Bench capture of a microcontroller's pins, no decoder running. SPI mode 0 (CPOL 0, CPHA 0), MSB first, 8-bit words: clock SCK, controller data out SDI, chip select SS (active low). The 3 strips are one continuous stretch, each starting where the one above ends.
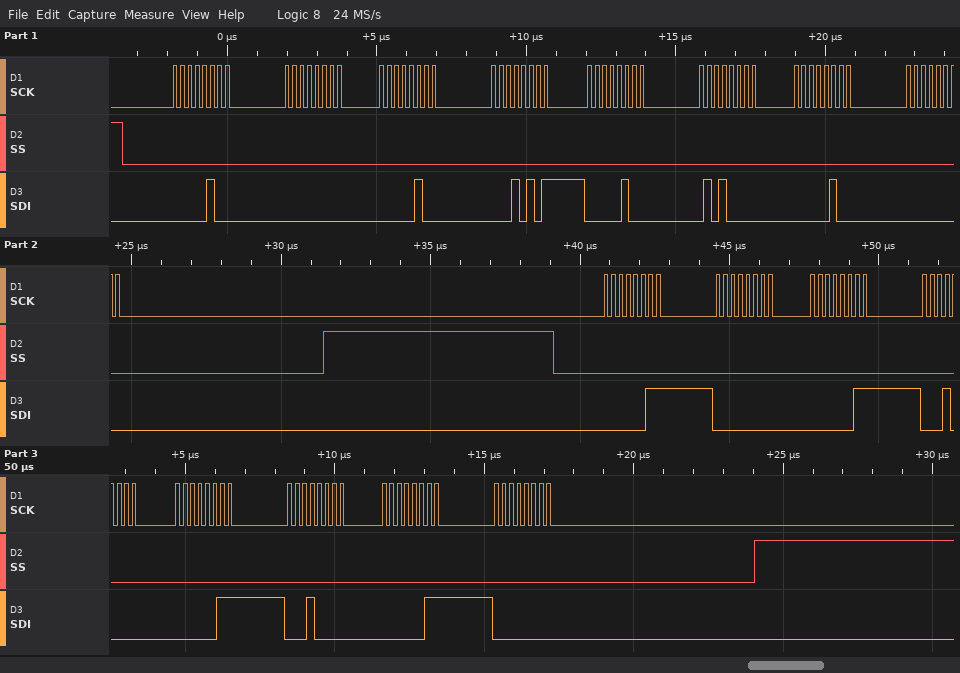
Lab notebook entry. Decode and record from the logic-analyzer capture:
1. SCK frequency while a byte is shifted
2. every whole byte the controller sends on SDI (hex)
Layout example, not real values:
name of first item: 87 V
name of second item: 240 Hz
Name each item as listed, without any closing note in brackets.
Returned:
SCK frequency while a byte is shifted: 4 MHz
every whole byte the controller sends on SDI: 04 00 04 15 04 50 04 00 03 00 03 10 03 10 03 00
